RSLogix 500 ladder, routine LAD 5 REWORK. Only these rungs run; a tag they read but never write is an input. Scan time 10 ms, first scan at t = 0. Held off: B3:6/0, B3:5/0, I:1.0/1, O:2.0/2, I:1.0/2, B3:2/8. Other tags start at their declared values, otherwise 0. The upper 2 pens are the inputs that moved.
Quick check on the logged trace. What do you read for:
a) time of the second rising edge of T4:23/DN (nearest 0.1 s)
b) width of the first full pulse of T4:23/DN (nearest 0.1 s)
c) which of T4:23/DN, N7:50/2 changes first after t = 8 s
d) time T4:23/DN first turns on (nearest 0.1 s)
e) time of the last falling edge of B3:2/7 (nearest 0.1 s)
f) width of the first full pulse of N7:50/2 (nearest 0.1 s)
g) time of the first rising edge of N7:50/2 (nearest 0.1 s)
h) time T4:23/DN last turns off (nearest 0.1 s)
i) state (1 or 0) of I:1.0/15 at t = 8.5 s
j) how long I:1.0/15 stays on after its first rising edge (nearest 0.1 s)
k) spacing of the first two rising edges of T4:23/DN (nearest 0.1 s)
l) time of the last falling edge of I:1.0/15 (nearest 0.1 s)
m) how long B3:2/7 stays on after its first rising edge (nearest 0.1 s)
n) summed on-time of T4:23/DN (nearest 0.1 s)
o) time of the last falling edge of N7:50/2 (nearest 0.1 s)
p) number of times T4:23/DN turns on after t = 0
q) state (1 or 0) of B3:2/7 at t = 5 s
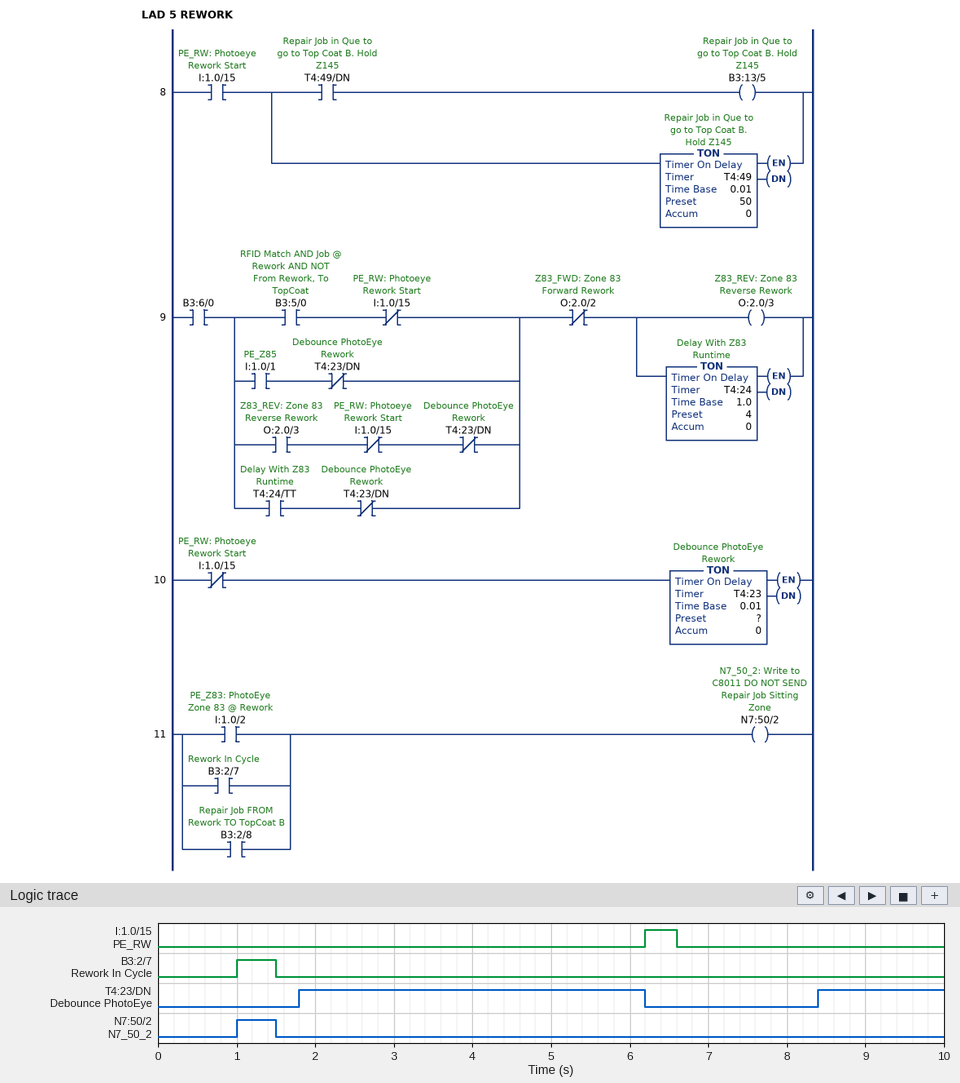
8.4 s
4.4 s
T4:23/DN
1.8 s
1.5 s
0.5 s
1.0 s
6.2 s
0
0.4 s
6.6 s
6.6 s
0.5 s
6.0 s
1.5 s
2
0
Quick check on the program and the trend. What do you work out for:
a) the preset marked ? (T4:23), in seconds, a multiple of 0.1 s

1.8 s
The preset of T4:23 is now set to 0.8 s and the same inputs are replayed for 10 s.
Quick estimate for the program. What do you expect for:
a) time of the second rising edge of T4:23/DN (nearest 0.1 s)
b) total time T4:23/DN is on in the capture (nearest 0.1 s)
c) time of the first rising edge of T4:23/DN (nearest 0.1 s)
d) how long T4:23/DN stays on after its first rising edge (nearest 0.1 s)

7.4 s
8.0 s
0.8 s
5.4 s
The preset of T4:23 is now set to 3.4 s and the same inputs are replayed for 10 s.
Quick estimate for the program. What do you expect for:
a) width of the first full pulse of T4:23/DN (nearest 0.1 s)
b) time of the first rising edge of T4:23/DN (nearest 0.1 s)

2.8 s
3.4 s
